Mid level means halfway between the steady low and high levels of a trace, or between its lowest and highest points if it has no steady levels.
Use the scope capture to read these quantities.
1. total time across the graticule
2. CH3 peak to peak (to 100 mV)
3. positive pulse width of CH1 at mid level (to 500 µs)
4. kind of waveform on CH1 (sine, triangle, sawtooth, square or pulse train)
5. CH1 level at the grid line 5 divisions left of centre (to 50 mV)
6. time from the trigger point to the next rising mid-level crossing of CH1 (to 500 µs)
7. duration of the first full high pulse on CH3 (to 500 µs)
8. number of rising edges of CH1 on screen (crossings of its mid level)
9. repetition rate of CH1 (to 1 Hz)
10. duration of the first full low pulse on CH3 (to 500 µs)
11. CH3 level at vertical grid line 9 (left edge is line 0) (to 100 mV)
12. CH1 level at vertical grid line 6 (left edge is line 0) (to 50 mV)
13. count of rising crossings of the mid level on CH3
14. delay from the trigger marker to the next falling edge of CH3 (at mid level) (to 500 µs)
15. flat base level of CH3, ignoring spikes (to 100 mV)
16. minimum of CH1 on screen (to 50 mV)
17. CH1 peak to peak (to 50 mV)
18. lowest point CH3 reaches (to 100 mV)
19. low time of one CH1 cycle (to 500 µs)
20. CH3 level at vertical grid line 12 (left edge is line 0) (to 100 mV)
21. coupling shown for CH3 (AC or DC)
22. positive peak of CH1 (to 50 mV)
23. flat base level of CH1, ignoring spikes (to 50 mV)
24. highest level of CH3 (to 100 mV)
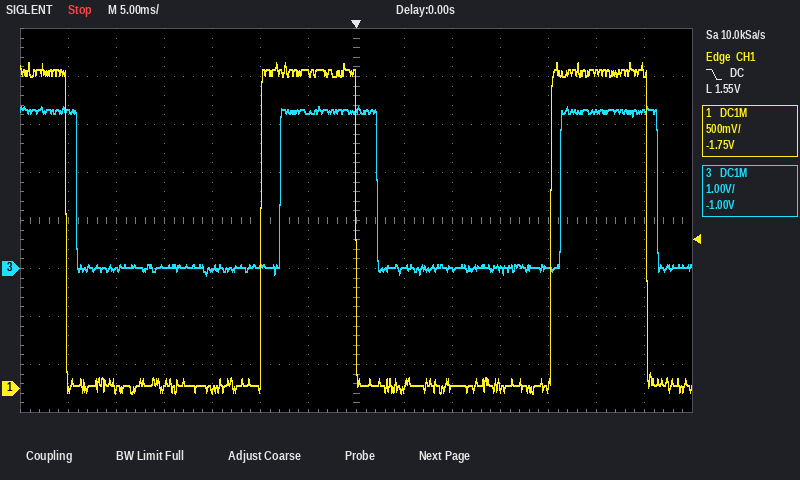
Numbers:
70 ms
3.5 V
10.0 ms
pulse train
0 mV
20.5 ms
10.0 ms
2
33 Hz
21.0 ms
0.0 V
3.30 V
2
2.0 ms
0.0 V
-50 mV
3.45 V
-100 mV
20.5 ms
3.3 V
DC
3.40 V
50 mV
3.4 V
